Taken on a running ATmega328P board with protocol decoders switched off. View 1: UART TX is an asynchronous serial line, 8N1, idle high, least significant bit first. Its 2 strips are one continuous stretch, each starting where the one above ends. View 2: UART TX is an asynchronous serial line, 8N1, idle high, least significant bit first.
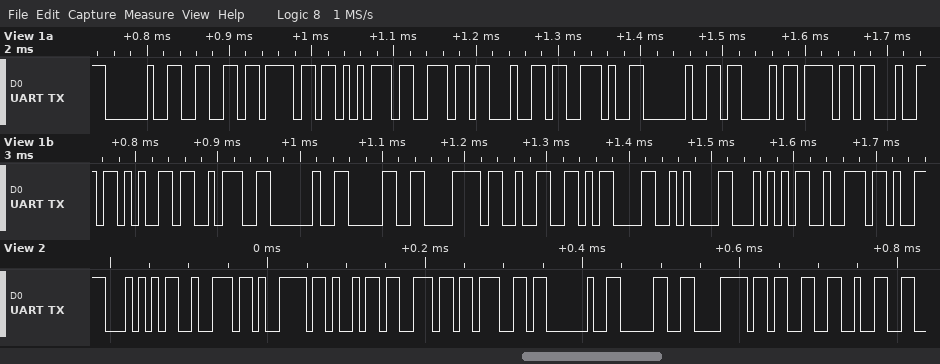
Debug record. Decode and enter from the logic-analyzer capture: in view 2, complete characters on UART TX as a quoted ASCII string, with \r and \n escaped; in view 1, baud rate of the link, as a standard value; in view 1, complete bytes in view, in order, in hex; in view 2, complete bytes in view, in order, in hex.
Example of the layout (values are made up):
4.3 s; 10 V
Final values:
"Trying 0x32"; 115200 baud; 20 66 6F 75 6E 64 2E 20 43 6F 64 65 3A 20 30 78 32 0D 0A 54 72; 54 72 79 69 6E 67 20 30 78 33 32
